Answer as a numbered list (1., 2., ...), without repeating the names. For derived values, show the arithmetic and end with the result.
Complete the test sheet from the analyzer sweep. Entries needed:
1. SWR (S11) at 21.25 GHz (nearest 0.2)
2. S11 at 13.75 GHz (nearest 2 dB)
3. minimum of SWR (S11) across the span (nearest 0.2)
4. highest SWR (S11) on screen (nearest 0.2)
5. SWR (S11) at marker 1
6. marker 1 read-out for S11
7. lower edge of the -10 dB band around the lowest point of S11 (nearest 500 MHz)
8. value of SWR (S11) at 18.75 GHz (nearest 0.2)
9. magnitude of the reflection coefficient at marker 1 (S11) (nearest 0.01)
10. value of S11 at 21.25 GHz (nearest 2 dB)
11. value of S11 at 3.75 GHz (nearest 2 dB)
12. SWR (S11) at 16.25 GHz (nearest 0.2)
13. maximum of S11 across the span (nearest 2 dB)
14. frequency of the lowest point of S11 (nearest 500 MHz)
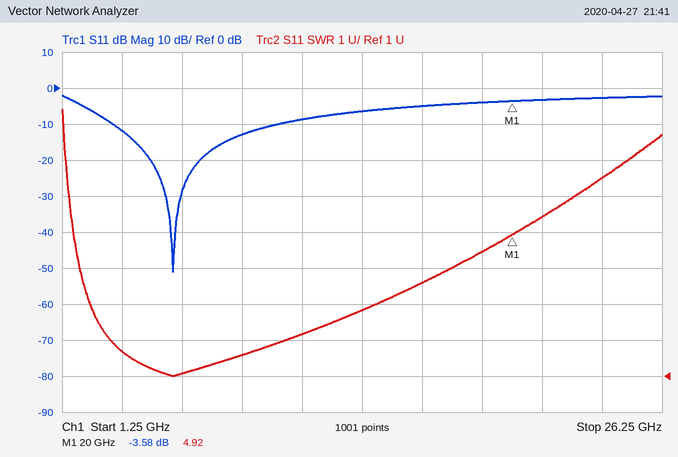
1. 5.4
2. -6 dB
3. 1.0
4. 8.4
5. 4.92
6. -3.58 dB
7. 3.5 GHz
8. 4.4
9. 10^(-3.58/20) ≈ 0.66
10. -4 dB
11. -12 dB
12. 3.6
13. -2 dB
14. 6.0 GHz
